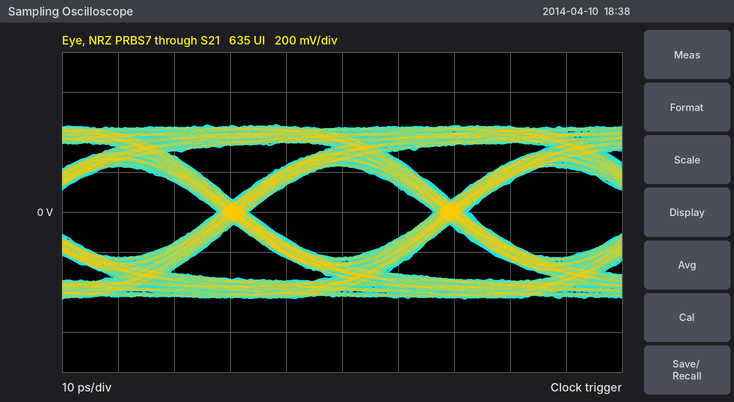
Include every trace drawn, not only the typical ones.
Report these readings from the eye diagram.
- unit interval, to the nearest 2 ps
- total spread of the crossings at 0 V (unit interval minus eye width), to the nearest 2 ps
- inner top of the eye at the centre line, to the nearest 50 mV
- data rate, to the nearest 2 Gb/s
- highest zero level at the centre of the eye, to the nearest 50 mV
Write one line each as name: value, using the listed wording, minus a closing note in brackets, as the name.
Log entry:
unit interval, to the nearest 2 ps: 38 ps
total spread of the crossings at 0 V (unit interval minus eye width), to the nearest 2 ps: 6 ps
inner top of the eye at the centre line, to the nearest 50 mV: 250 mV
data rate, to the nearest 2 Gb/s: 26 Gb/s
highest zero level at the centre of the eye, to the nearest 50 mV: -250 mV
